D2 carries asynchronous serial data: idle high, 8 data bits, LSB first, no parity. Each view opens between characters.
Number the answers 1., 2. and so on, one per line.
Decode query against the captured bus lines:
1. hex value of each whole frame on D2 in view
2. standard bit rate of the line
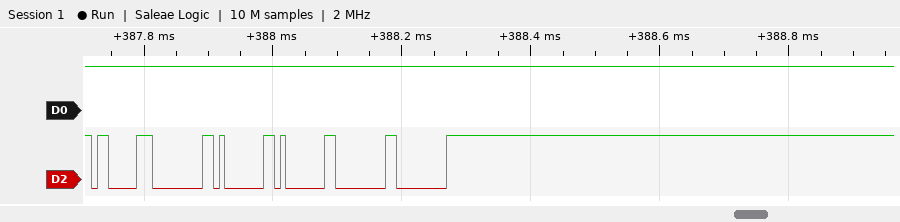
1. 83, 00, 01, 01, 00, 00
2. 115200 baud
